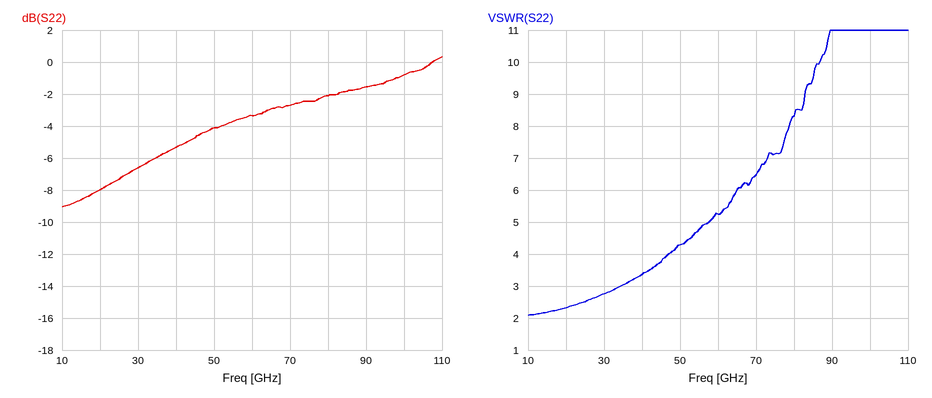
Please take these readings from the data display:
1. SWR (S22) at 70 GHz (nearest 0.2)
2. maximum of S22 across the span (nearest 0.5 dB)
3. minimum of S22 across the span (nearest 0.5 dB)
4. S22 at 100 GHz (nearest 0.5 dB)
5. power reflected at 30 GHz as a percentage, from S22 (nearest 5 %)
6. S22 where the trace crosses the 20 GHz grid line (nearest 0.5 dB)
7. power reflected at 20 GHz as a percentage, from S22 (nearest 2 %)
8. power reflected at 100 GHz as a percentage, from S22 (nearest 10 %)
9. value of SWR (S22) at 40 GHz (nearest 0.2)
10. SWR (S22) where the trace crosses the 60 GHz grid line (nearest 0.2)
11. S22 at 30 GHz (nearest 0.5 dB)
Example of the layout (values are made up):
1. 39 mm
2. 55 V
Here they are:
1. 6.4
2. 0.5 dB
3. -9.0 dB
4. -1.0 dB
5. 20 %
6. -8.0 dB
7. 16 %
8. 80 %
9. 3.4
10. 5.2
11. -6.5 dB
